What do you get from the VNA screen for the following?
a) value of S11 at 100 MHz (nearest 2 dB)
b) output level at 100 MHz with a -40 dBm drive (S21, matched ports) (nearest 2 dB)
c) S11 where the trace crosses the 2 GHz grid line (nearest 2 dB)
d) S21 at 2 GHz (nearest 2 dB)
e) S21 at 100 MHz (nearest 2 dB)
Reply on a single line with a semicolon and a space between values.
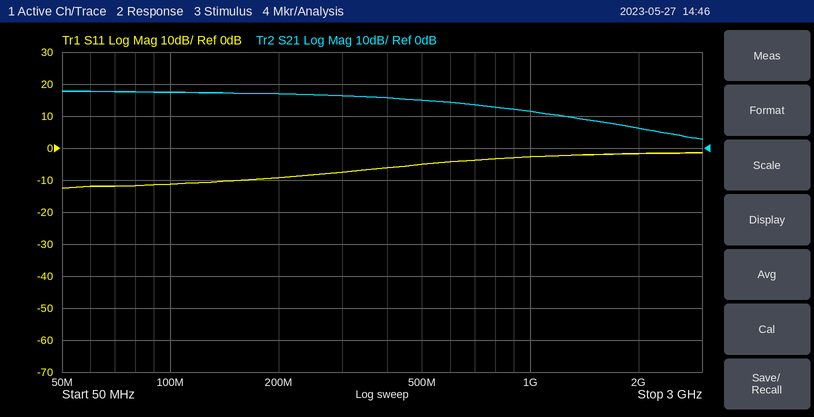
-12 dB; -22 dBm; -2 dB; 6 dB; 18 dB
